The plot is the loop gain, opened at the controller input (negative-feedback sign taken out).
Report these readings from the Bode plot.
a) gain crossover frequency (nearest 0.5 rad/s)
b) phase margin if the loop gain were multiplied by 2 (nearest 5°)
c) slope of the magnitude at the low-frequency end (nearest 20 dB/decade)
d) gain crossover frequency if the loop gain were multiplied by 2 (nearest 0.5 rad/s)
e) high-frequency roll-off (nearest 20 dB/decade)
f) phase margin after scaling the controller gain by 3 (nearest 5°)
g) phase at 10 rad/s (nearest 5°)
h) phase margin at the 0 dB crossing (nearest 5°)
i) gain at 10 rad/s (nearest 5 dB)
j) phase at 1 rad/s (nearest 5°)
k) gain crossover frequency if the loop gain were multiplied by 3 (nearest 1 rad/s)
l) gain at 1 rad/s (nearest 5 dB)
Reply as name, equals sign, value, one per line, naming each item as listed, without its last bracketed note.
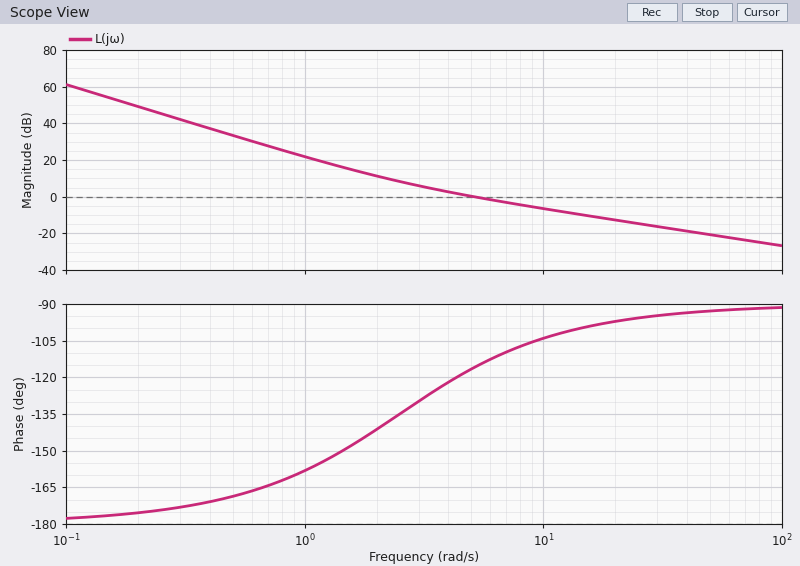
gain crossover frequency = 5.0 rad/s
phase margin if the loop gain were multiplied by 2 = 75°
slope of the magnitude at the low-frequency end = -40 dB/decade
gain crossover frequency if the loop gain were multiplied by 2 = 9.5 rad/s
high-frequency roll-off = -20 dB/decade
phase margin after scaling the controller gain by 3 = 80°
phase at 10 rad/s = -105°
phase margin at the 0 dB crossing = 65°
gain at 10 rad/s = -5 dB
phase at 1 rad/s = -160°
gain crossover frequency if the loop gain were multiplied by 3 = 14 rad/s
gain at 1 rad/s = 20 dB
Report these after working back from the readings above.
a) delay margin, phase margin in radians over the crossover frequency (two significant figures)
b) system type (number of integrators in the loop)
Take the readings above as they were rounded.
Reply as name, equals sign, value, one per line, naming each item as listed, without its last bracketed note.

delay margin, phase margin in radians over the crossover frequency = 0.23 s
system type = 2
